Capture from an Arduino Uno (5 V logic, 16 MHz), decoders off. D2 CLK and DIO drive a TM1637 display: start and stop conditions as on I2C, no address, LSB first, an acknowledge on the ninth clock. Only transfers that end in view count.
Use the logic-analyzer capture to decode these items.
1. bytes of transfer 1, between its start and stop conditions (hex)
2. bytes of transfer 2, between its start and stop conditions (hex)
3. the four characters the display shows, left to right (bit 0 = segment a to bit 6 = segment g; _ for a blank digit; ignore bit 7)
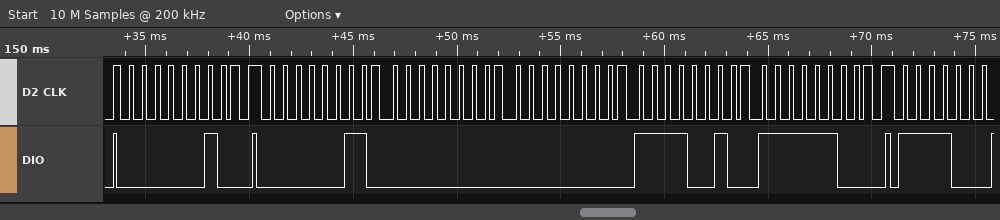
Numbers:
40
C0 00 00 4F 3F
__30
